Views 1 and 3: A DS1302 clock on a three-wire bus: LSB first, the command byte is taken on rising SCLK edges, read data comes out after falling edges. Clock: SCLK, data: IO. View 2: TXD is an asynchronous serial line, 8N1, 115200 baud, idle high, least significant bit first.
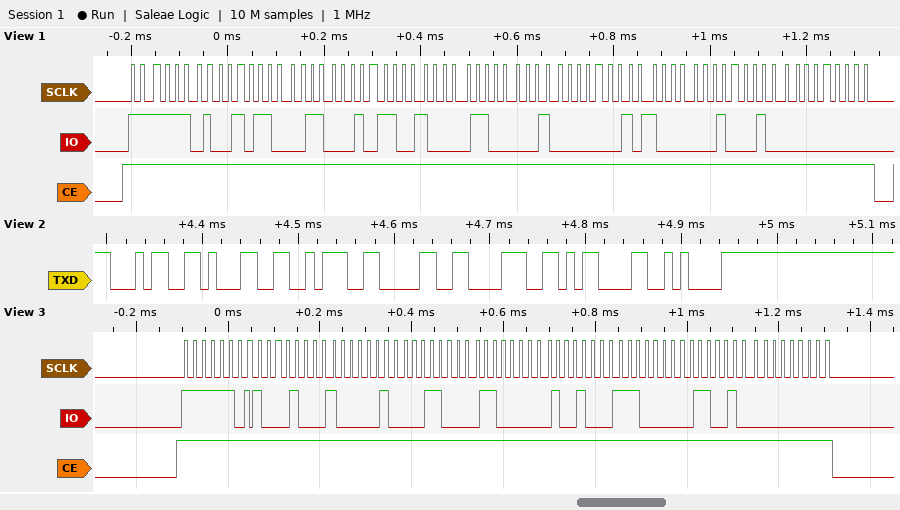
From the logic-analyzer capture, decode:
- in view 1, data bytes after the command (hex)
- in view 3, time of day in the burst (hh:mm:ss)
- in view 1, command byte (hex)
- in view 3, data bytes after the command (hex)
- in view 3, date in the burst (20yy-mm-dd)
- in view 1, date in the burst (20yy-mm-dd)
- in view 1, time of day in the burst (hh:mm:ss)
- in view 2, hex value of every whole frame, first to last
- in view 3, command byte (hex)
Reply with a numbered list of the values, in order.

1. 34 46 13 06 01 05 22 00
2. 18:41:11
3. 0xBF
4. 11 41 18 06 12 07 26 00
5. 2026-12-06
6. 2022-01-06
7. 13:46:34
8. 0x34 0x31 0x3A 0x30 0x38 0x0D 0x0A
9. 0xBF
